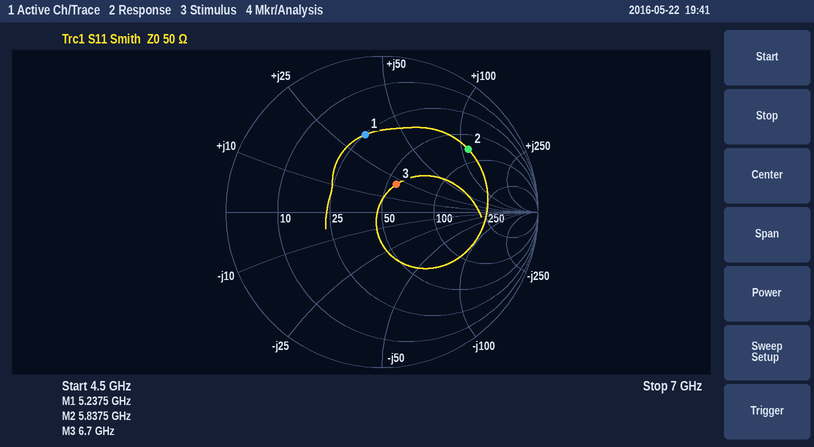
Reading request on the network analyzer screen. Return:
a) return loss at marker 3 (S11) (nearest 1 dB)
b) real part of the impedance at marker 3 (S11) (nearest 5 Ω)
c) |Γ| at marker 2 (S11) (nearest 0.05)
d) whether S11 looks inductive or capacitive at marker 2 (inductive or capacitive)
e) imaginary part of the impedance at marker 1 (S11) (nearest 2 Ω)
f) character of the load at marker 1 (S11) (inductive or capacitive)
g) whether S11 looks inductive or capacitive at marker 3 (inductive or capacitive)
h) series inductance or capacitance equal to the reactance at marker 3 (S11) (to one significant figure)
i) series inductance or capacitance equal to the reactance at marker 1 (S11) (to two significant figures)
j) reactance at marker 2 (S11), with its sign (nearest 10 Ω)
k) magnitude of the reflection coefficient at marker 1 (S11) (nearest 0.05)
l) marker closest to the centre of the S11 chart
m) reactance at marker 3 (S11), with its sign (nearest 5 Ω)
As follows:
14 dB
55 Ω
0.70
inductive
+34 Ω
inductive
inductive
500 pH
1.0 nH
+110 Ω
0.50
marker 3
+20 Ω
